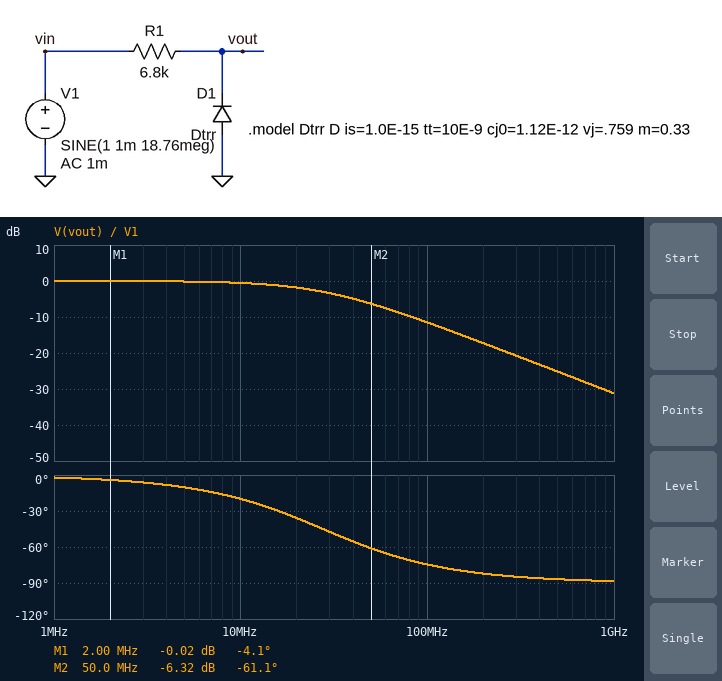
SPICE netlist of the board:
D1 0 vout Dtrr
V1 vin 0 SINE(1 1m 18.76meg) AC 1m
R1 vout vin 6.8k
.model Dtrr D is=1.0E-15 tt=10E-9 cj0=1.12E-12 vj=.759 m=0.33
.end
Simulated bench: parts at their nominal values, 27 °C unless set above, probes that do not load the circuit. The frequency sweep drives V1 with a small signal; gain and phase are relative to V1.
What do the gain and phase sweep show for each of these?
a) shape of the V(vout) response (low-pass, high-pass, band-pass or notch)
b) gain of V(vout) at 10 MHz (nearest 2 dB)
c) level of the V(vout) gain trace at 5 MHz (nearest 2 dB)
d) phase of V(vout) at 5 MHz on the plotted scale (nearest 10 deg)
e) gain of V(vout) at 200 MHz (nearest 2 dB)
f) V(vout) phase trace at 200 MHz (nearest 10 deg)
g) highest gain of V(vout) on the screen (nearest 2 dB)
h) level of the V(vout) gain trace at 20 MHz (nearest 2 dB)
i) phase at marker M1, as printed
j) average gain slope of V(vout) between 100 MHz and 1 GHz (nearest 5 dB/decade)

low-pass
0 dB
0 dB
-10 deg
-18 dB
-80 deg
0 dB
-2 dB
-4.1 deg
-20 dB/decade
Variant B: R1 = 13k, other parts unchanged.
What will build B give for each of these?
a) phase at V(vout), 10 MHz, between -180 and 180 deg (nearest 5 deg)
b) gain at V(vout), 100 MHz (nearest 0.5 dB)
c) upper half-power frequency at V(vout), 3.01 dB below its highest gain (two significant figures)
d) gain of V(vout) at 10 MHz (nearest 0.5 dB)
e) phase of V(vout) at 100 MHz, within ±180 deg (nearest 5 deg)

-35 deg
-17.0 dB
14 MHz
-1.5 dB
-80 deg
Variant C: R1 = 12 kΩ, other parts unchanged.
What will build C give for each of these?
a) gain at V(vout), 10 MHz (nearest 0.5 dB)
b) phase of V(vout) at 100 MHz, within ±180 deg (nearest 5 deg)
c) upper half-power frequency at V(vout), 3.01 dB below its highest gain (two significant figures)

-1.5 dB
-80 deg
16 MHz
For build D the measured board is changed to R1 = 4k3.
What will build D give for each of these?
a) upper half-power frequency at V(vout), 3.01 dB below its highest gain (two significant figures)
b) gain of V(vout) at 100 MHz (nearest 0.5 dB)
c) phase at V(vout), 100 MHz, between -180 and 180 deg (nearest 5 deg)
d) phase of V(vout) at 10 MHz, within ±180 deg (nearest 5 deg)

44 MHz
-8.0 dB
-65 deg
-15 deg
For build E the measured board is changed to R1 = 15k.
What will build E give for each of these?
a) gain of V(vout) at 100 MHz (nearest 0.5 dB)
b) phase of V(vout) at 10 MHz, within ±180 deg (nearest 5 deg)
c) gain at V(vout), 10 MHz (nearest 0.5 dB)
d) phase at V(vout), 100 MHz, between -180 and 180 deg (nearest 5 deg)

-18.0 dB
-40 deg
-2.0 dB
-85 deg
